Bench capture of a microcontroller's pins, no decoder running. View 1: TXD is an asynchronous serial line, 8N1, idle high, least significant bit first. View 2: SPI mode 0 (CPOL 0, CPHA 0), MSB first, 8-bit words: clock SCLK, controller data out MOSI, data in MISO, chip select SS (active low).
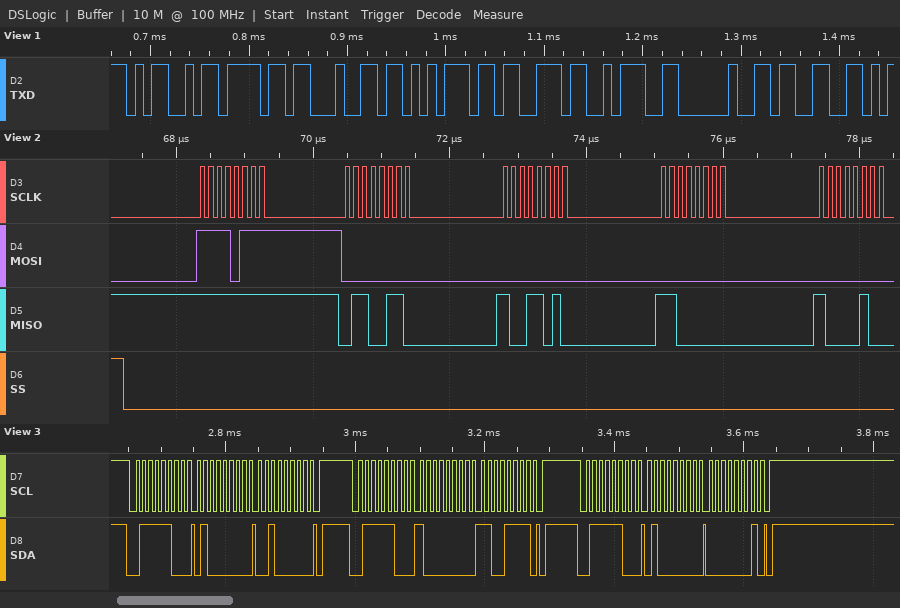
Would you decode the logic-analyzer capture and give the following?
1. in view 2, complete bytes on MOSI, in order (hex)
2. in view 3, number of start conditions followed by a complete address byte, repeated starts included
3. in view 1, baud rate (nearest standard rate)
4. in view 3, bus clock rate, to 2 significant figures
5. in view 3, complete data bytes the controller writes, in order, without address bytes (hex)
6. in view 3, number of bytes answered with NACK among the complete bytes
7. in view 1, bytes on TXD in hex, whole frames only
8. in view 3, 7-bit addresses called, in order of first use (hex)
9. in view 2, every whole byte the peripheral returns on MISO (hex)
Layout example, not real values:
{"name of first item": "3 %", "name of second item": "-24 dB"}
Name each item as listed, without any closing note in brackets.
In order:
{"in view 2, complete bytes on MOSI, in order": "F7 00 00 00 00", "in view 3, number of start conditions followed by a complete address byte, repeated starts included": "3", "in view 1, baud rate": "115200 baud", "in view 3, bus clock rate, to 2 significant figures": "100 kHz", "in view 3, complete data bytes the controller writes, in order, without address bytes": "40 20 80 CF 40 01", "in view 3, number of bytes answered with NACK among the complete bytes": "0", "in view 1, bytes on TXD in hex, whole frames only": "0x4D 0x6F 0x64 0x75 0x73 0x3A 0x20 0x33", "in view 3, 7-bit addresses called, in order of first use": "0x3E", "in view 2, every whole byte the peripheral returns on MISO": "FF 66 9A C0 84"}
